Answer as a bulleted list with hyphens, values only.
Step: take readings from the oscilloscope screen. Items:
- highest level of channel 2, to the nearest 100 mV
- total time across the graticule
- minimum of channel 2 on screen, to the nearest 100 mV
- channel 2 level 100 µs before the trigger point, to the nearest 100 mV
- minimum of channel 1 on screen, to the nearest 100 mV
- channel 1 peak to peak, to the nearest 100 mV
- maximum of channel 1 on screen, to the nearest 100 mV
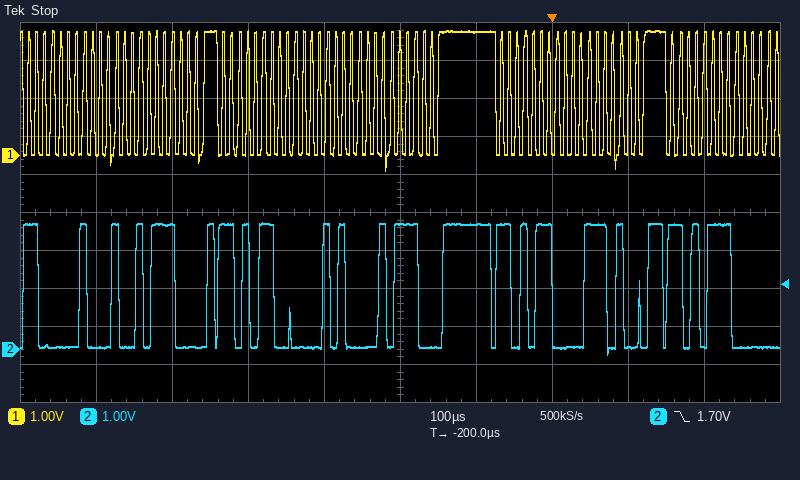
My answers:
- 3.3 V
- 1 ms
- -100 mV
- 3.3 V
- -400 mV
- 3.7 V
- 3.3 V
